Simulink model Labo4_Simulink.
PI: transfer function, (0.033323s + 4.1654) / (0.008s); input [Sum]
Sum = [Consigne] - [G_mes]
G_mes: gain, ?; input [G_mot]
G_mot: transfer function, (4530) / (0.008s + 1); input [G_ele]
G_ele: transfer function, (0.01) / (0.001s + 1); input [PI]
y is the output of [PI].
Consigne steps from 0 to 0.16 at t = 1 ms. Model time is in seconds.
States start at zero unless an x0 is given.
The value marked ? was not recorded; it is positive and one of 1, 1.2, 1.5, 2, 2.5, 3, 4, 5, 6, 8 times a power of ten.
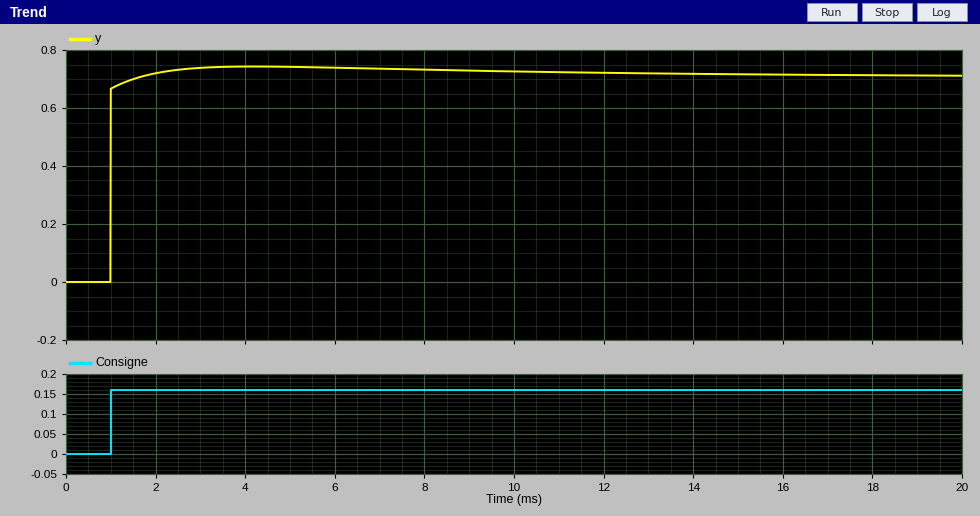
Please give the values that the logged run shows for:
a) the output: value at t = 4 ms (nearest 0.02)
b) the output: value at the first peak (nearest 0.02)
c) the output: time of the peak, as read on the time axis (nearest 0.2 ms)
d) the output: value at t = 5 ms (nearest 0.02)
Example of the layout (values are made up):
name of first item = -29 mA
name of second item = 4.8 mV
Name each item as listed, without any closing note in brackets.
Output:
the output: value at t = 4 ms = 0.74
the output: value at the first peak = 0.74
the output: time of the peak, as read on the time axis = 4.2 ms
the output: value at t = 5 ms = 0.74
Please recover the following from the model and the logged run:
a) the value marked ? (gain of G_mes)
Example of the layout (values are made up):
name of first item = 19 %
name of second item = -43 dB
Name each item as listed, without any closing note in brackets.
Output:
the value marked ? = 0.005
